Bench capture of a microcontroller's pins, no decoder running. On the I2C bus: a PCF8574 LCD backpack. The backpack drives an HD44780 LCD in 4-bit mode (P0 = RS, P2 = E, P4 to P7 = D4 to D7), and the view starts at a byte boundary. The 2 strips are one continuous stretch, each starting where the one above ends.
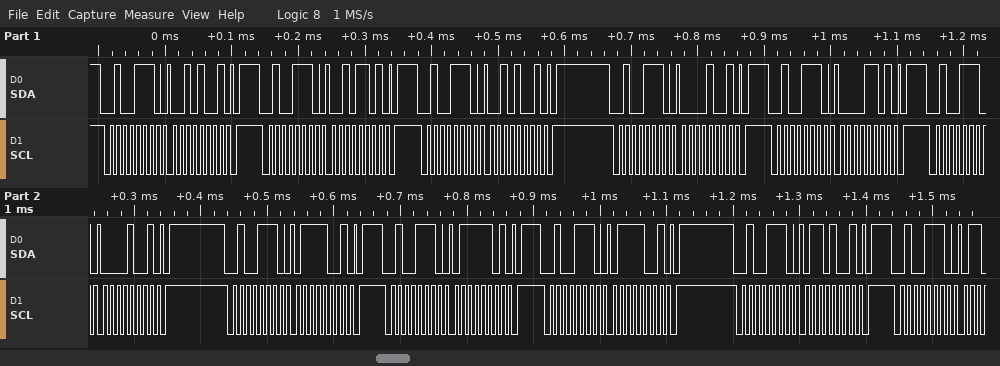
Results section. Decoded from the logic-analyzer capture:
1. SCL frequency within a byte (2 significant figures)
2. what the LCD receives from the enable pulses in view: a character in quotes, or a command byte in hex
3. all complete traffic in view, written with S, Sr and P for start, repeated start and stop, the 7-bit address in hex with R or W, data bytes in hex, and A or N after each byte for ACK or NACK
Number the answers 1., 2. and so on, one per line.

1. 100 kHz
2. ' '
3. S 27W A 29 A P S 27W A 2D A P S 27W A 29 A P S 27W A 09 A P S 27W A 0D A P S 27W A 09 A P S 27W A 79 A P S 27W A 7D A P S 27W A 79 A P S 27W A 69 A P S 27W A
